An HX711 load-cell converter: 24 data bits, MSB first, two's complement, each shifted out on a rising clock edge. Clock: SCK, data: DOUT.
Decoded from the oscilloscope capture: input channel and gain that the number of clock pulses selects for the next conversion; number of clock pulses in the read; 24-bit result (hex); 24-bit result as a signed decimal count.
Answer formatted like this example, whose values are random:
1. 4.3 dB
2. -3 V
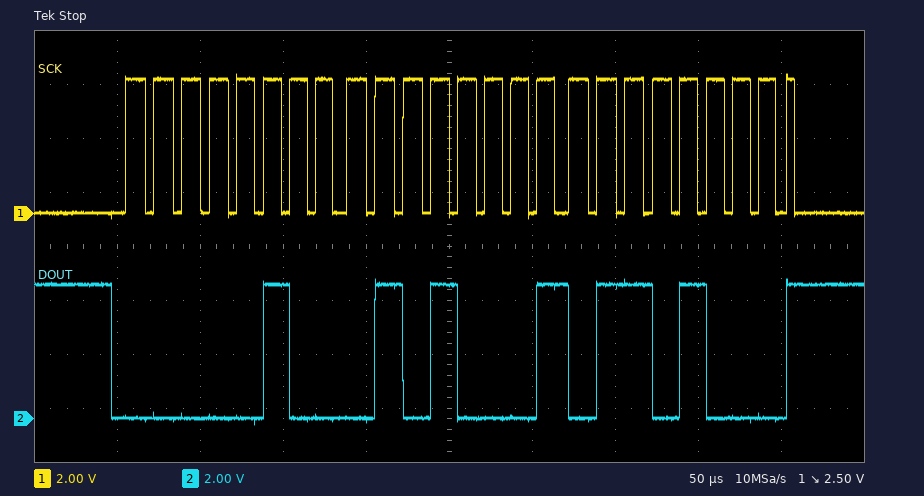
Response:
1. channel A, gain 128
2. 25
3. 0x045168
4. 282984
